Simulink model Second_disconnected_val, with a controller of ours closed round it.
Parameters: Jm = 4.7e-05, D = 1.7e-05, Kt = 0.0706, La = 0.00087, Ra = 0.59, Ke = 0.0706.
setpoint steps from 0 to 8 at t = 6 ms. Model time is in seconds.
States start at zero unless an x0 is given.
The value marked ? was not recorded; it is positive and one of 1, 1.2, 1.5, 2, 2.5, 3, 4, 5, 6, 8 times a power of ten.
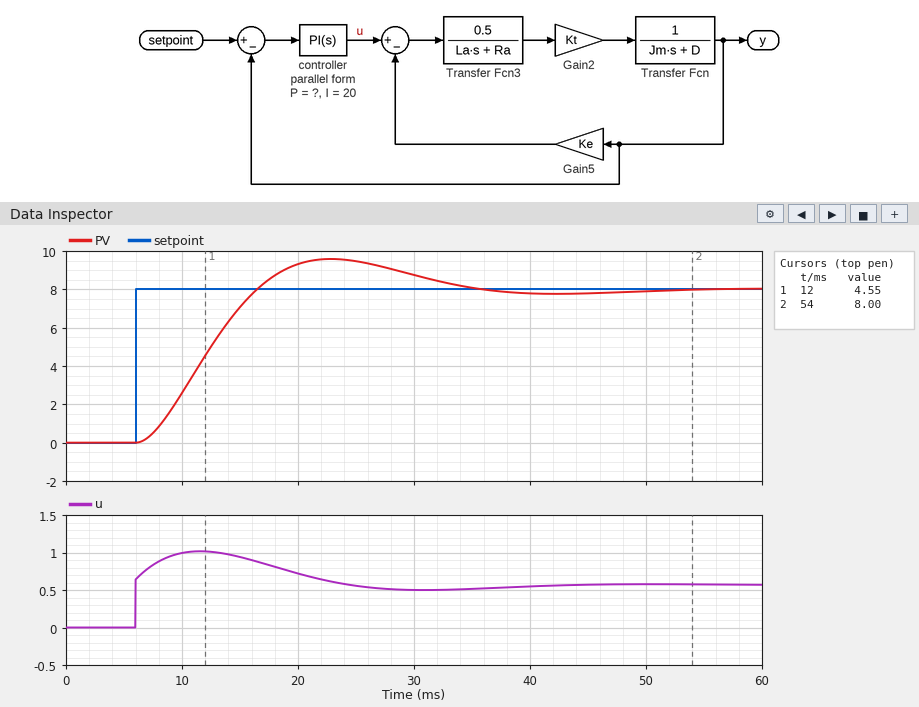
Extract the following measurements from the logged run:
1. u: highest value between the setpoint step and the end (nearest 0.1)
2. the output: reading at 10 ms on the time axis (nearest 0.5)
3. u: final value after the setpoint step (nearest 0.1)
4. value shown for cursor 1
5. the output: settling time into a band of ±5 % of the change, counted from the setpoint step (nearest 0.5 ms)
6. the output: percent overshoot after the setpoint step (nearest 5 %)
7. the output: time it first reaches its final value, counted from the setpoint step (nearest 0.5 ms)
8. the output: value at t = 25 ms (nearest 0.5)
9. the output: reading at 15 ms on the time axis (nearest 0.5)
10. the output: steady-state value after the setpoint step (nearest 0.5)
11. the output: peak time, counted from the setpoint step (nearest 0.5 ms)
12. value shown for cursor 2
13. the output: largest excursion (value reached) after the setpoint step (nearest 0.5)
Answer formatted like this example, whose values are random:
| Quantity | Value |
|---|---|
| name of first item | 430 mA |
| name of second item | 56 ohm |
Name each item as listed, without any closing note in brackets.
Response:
| Quantity | Value |
|---|---|
| u: highest value between the setpoint step and the end | 1.0 |
| the output: reading at 10 ms on the time axis | 2.5 |
| u: final value after the setpoint step | 0.6 |
| value shown for cursor 1 | 4.55 |
| the output: settling time into a band of ±5 % of the change, counted from the setpoint step | 26.5 ms |
| the output: percent overshoot after the setpoint step | 20 % |
| the output: time it first reaches its final value, counted from the setpoint step | 10.5 ms |
| the output: value at t = 25 ms | 9.5 |
| the output: reading at 15 ms on the time axis | 7.0 |
| the output: steady-state value after the setpoint step | 8.0 |
| the output: peak time, counted from the setpoint step | 17.0 ms |
| value shown for cursor 2 | 8.00 |
| the output: largest excursion (value reached) after the setpoint step | 9.5 |
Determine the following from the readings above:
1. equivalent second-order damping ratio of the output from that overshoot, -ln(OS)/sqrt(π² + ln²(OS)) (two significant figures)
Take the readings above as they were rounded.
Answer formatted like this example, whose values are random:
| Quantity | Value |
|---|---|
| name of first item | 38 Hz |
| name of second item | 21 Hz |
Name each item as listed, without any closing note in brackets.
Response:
| Quantity | Value |
|---|---|
| equivalent second-order damping ratio of the output from that overshoot, -ln(OS)/sqrt(π² + ln²(OS)) | 0.46 |
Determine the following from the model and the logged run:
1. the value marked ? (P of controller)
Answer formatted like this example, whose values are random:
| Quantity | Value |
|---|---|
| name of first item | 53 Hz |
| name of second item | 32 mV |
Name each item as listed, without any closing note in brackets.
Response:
| Quantity | Value |
|---|---|
| the value marked ? | 0.08 |
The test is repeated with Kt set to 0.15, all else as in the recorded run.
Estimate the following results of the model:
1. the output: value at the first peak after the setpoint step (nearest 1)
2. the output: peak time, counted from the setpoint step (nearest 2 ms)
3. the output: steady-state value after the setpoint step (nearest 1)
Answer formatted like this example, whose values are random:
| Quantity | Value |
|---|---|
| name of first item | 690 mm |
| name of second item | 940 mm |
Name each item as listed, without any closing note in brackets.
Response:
| Quantity | Value |
|---|---|
| the output: value at the first peak after the setpoint step | 8 |
| the output: peak time, counted from the setpoint step | 10 ms |
| the output: steady-state value after the setpoint step | 8 |
